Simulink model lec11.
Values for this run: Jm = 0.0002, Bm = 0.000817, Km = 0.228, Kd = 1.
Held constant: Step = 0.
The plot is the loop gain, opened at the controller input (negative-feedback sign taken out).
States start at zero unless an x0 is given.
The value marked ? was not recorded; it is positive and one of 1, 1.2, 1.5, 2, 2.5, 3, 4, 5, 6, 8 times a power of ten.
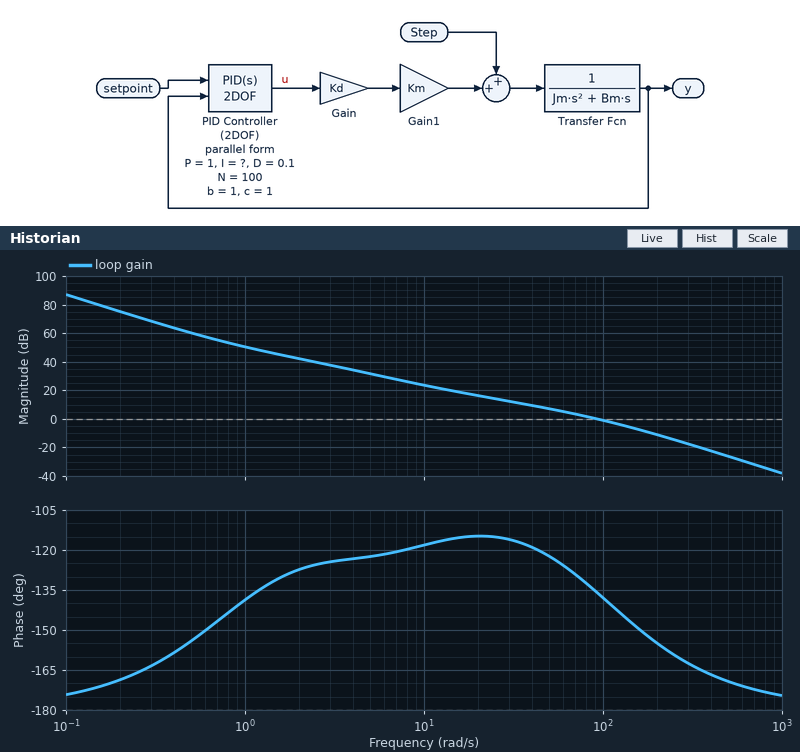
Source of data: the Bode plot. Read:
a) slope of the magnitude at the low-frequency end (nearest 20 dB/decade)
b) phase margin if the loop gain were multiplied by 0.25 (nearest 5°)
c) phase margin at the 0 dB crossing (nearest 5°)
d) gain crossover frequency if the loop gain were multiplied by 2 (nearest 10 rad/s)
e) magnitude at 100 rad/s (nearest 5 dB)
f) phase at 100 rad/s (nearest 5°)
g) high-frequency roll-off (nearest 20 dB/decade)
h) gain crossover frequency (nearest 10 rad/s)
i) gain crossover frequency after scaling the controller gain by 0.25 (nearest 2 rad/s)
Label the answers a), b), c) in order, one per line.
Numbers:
a) -40 dB/decade
b) 65°
c) 45°
d) 140 rad/s
e) 0 dB
f) -140°
g) -40 dB/decade
h) 90 rad/s
i) 30 rad/s
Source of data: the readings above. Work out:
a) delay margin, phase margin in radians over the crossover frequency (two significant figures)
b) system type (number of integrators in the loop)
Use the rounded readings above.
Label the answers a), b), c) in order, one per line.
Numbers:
a) 0.0087 s
b) 2
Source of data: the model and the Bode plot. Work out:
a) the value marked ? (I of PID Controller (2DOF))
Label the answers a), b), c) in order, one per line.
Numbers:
a) 0.8
